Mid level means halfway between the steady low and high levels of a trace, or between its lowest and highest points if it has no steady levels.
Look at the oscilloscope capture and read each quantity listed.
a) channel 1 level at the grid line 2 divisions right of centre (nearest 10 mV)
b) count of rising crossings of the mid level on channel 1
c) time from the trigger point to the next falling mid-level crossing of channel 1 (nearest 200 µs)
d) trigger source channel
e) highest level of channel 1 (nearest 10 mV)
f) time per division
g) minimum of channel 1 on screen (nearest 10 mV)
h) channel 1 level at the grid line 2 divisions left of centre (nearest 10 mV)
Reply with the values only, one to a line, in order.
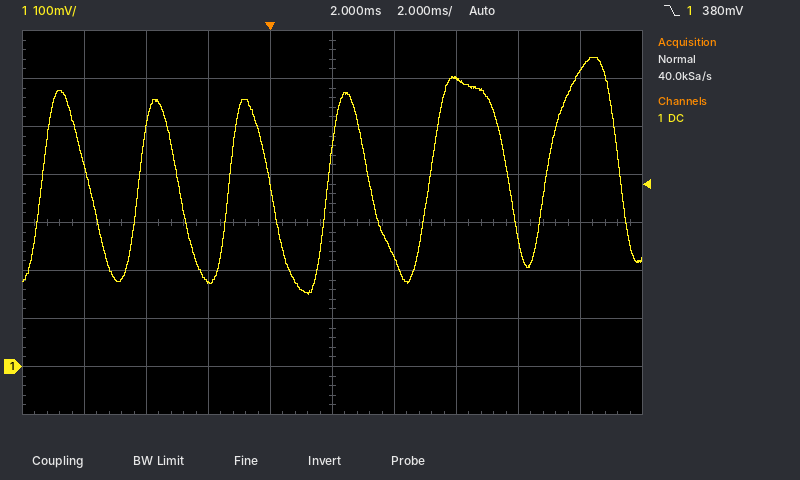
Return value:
600 mV
6
3.2 ms
channel 1
640 mV
2 ms
150 mV
180 mV
